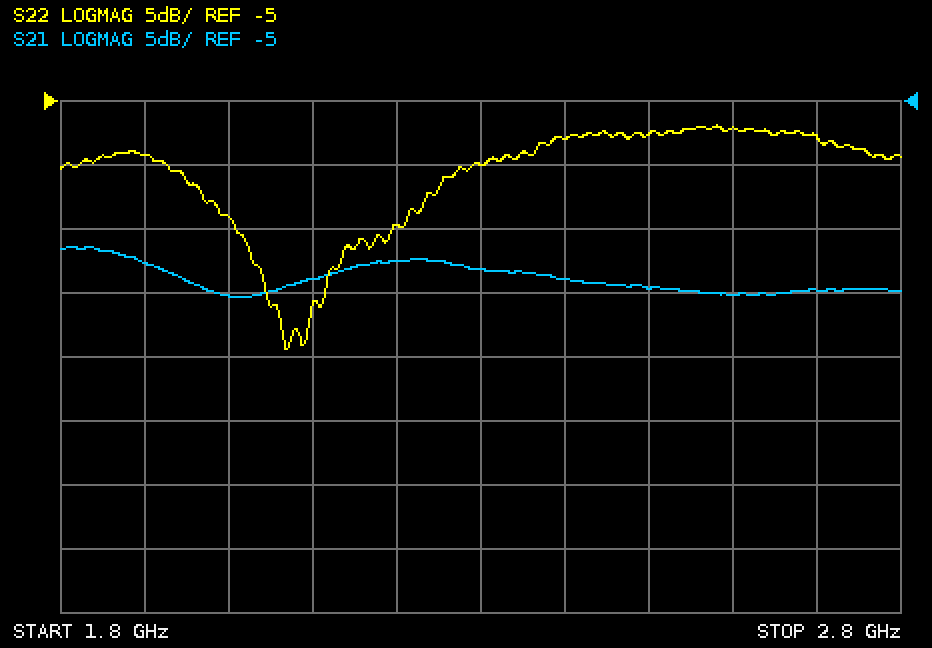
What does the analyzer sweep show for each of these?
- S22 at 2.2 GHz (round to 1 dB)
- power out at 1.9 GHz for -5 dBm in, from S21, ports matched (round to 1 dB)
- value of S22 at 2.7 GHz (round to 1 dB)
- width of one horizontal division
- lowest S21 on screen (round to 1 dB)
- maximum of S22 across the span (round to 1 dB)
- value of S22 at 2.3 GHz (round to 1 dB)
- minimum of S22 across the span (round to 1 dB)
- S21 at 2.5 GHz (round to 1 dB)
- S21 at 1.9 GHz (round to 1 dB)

-15 dB
-23 dBm
-8 dB
100 MHz
-20 dB
-7 dB
-10 dB
-24 dB
-20 dB
-18 dB
